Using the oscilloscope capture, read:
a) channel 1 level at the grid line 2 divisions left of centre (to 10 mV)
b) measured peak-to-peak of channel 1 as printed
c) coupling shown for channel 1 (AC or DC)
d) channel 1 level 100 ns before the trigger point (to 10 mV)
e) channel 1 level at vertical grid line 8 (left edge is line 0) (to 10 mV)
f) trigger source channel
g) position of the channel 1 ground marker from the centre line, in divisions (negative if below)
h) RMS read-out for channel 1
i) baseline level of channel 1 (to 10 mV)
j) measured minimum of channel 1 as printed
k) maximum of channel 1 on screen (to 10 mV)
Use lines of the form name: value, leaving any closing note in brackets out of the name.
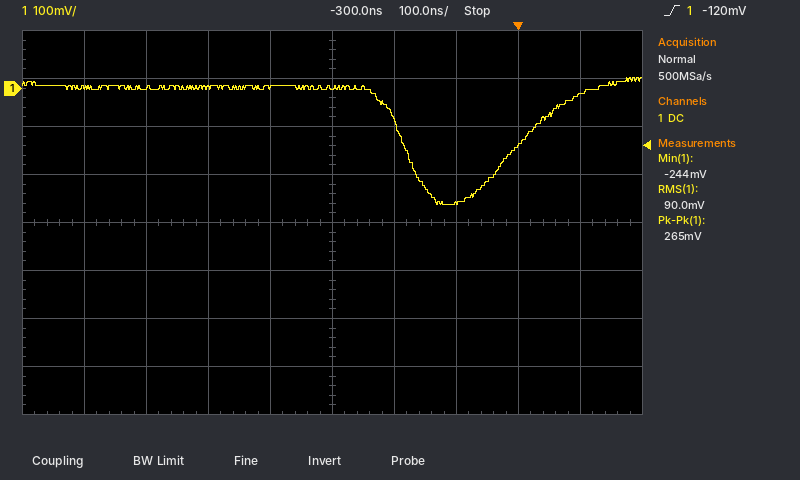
channel 1 level at the grid line 2 divisions left of centre: 0 mV
measured peak-to-peak of channel 1 as printed: 265 mV
coupling shown for channel 1: DC
channel 1 level 100 ns before the trigger point: -240 mV
channel 1 level at vertical grid line 8 (left edge is line 0): -120 mV
trigger source channel: channel 1
position of the channel 1 ground marker from the centre line, in divisions: +2.8 div
RMS read-out for channel 1: 90.0 mV
baseline level of channel 1: 0 mV
measured minimum of channel 1 as printed: -244 mV
maximum of channel 1 on screen: 20 mV
